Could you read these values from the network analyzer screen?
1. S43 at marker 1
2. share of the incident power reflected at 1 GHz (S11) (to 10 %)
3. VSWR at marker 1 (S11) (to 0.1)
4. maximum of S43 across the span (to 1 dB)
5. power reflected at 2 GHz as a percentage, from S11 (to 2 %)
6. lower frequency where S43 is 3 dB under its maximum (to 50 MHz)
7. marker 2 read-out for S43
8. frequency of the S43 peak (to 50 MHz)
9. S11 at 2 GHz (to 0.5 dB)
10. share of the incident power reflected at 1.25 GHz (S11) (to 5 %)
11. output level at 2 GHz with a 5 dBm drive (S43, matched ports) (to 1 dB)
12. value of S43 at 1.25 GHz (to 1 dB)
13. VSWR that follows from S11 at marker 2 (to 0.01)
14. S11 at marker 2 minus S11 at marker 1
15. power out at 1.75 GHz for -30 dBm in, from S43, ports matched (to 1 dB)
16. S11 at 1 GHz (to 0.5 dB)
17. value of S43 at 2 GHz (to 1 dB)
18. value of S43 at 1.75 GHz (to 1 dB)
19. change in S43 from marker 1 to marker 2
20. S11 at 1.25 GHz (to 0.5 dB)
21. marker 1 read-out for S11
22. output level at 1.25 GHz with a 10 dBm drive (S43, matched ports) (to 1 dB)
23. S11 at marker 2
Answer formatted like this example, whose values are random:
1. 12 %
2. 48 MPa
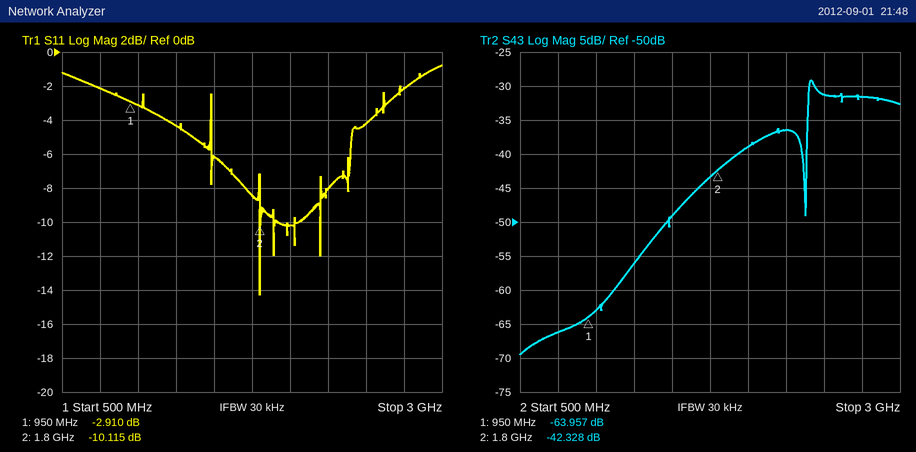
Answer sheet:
1. -63.957 dB
2. 50 %
3. 6.0
4. -29 dB
5. 10 %
6. 2.40 GHz
7. -42.328 dB
8. 2.40 GHz
9. -10.0 dB
10. 35 %
11. -34 dBm
12. -56 dB
13. 1.91
14. -7.205 dB
15. -73 dBm
16. -3.0 dB
17. -39 dB
18. -43 dB
19. 21.629 dB
20. -4.5 dB
21. -2.910 dB
22. -46 dBm
23. -10.115 dB
